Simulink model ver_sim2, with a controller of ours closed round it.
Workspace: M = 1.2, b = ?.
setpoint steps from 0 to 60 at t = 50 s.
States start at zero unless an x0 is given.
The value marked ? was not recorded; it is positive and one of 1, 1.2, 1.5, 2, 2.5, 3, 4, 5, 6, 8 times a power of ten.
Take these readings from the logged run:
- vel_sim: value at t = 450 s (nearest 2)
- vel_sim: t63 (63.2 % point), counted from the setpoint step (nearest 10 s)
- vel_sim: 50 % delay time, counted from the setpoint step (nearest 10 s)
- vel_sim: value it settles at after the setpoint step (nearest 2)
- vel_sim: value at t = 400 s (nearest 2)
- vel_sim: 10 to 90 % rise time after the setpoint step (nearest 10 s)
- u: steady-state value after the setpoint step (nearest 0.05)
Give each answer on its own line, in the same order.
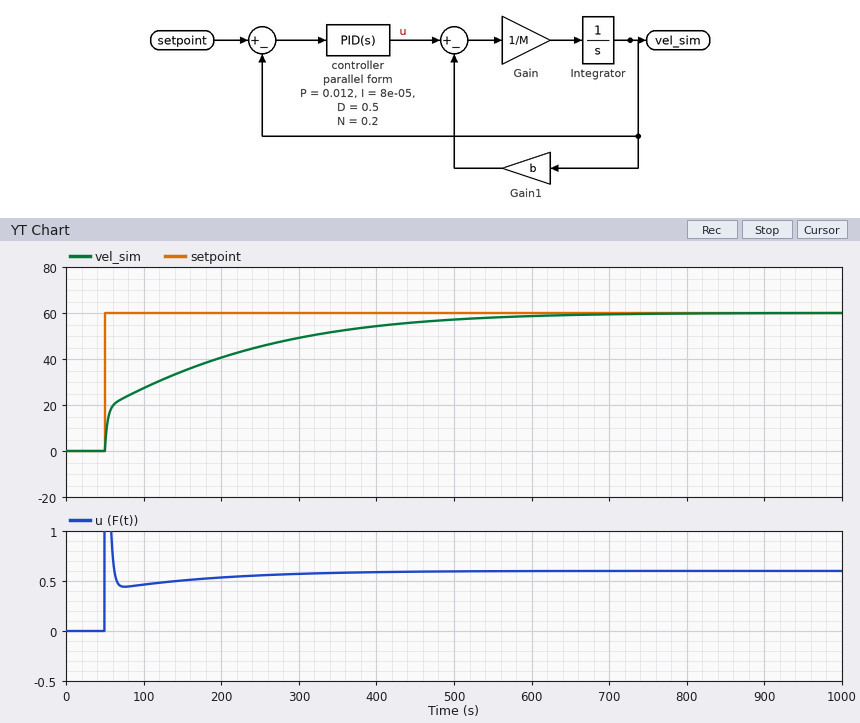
56
130 s
70 s
60
54
340 s
0.60
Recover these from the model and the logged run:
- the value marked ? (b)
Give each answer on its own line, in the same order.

0.01
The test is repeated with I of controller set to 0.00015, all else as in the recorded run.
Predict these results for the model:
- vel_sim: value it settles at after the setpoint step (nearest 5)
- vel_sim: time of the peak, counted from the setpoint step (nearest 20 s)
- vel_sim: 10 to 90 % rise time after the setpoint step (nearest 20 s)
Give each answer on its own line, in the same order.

60
400 s
200 s
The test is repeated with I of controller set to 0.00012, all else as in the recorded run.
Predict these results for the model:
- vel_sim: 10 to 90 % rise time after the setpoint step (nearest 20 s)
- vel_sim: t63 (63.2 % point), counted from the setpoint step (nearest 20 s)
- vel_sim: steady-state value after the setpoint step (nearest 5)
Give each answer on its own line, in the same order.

240 s
100 s
60
